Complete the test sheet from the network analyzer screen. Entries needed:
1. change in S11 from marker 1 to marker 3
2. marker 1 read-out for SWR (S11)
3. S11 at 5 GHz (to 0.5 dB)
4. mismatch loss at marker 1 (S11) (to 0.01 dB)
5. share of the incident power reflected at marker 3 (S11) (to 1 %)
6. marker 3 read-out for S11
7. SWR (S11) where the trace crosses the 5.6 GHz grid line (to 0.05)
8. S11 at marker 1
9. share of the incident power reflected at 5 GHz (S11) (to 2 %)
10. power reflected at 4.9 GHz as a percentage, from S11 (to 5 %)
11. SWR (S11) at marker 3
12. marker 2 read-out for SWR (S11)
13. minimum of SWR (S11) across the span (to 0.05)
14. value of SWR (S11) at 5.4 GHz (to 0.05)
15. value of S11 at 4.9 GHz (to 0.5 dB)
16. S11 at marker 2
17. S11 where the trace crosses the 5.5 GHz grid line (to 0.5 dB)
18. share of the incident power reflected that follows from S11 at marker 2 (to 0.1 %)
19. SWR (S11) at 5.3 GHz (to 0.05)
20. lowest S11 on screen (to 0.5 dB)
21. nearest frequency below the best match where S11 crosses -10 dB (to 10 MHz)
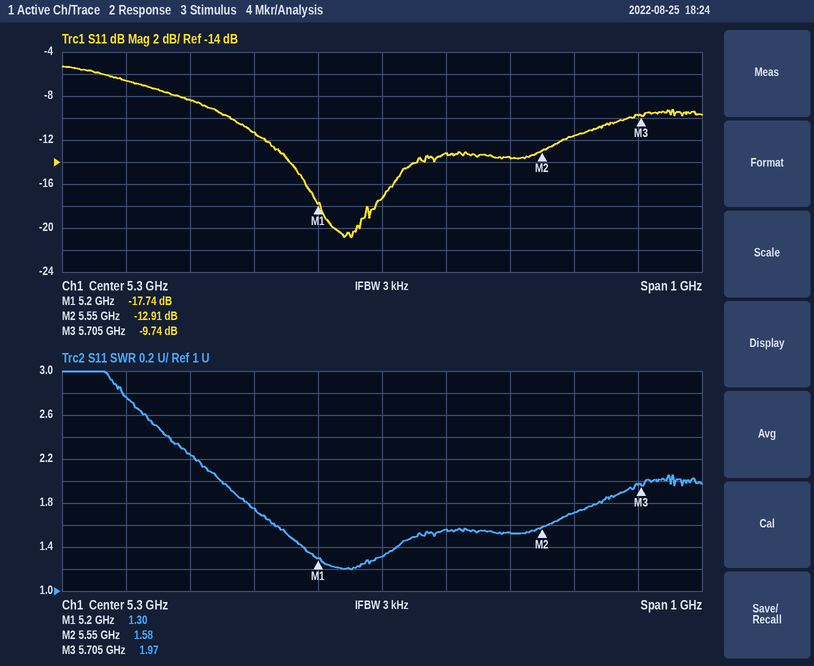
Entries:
8.00 dB
1.30
-8.5 dB
0.07 dB
11 %
-9.74 dB
1.70
-17.74 dB
14 %
20 %
1.97
1.58
1.20
1.55
-6.5 dB
-12.91 dB
-13.5 dB
5.1 %
1.30
-21.0 dB
5.06 GHz
